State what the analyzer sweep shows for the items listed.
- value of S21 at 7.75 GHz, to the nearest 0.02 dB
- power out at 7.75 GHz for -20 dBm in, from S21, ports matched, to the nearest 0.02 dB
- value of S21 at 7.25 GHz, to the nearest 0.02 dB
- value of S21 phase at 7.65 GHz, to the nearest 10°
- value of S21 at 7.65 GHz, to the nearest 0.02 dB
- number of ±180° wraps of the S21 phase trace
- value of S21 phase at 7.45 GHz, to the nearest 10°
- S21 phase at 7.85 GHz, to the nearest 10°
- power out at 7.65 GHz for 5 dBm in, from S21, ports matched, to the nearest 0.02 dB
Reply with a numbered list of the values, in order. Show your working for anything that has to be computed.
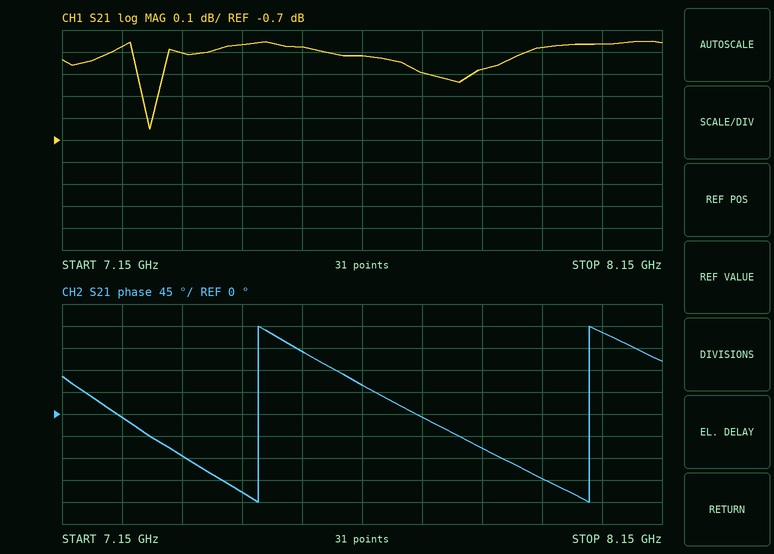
1. -0.40 dB
2. -20 dBm + (-0.40 dB) = -20.40 dBm
3. -0.28 dB
4. 60°
5. -0.32 dB
6. 2
7. -160°
8. -70°
9. 5 dBm + (-0.32 dB) = 4.68 dBm
